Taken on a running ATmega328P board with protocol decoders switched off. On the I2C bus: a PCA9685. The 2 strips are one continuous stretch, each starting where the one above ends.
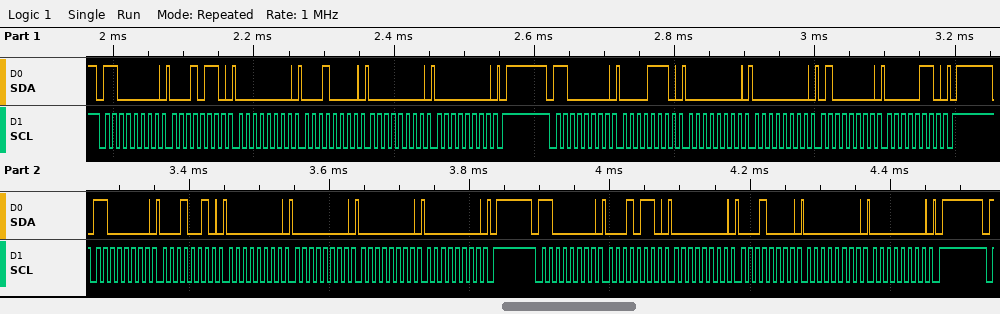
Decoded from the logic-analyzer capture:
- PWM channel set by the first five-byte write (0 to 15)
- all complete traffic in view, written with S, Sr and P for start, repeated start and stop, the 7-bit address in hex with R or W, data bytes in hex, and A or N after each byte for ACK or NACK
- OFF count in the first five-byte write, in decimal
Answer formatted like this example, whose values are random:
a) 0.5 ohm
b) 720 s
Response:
a) 4
b) S 60W A 16 A 00 A 10 A 00 A 00 A P S 60W A 0E A 00 A 00 A 40 A 06 A P S 60W A 12 A 00 A 00 A 00 A 00 A P S 60W A 16 A 00 A 10 A 00 A 00 A P
c) 0
